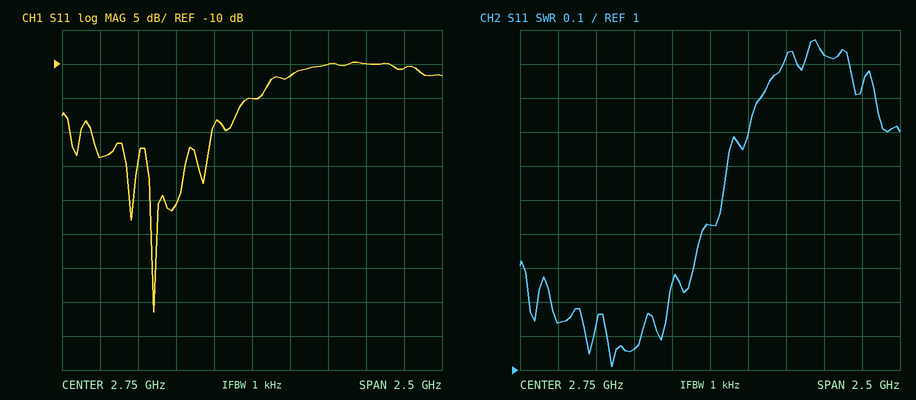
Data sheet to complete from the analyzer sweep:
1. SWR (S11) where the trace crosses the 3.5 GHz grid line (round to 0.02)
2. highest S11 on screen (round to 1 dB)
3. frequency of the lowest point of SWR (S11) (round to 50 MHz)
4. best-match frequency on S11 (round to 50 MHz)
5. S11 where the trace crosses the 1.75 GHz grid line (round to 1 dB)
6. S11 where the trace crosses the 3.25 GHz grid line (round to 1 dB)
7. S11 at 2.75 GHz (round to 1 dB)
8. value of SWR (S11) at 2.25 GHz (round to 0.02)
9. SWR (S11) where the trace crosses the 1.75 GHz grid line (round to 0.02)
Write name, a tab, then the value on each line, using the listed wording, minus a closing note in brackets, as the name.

SWR (S11) where the trace crosses the 3.5 GHz grid line	1.92
highest S11 on screen	-10 dB
frequency of the lowest point of SWR (S11)	2.10 GHz
best-match frequency on S11	2.10 GHz
S11 where the trace crosses the 1.75 GHz grid line	-24 dB
S11 where the trace crosses the 3.25 GHz grid line	-10 dB
S11 at 2.75 GHz	-15 dB
value of SWR (S11) at 2.25 GHz	1.06
SWR (S11) where the trace crosses the 1.75 GHz grid line	1.14
